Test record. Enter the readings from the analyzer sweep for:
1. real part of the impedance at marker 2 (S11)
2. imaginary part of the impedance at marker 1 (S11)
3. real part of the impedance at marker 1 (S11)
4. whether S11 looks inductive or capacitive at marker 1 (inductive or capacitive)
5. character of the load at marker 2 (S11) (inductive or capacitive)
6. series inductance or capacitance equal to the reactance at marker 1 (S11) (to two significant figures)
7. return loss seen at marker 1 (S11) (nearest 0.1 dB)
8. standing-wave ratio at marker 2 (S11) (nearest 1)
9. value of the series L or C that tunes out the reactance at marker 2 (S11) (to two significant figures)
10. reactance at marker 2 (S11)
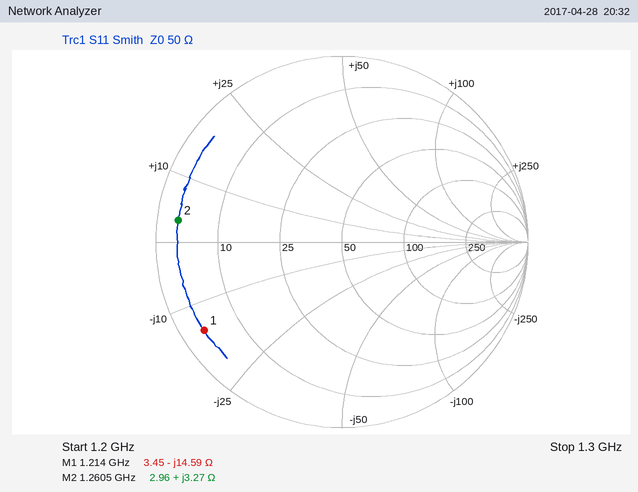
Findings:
2.96 Ω
-14.59 Ω
3.45 Ω
capacitive
inductive
9.0 pF
1.1 dB
17
39 pF
+3.27 Ω
